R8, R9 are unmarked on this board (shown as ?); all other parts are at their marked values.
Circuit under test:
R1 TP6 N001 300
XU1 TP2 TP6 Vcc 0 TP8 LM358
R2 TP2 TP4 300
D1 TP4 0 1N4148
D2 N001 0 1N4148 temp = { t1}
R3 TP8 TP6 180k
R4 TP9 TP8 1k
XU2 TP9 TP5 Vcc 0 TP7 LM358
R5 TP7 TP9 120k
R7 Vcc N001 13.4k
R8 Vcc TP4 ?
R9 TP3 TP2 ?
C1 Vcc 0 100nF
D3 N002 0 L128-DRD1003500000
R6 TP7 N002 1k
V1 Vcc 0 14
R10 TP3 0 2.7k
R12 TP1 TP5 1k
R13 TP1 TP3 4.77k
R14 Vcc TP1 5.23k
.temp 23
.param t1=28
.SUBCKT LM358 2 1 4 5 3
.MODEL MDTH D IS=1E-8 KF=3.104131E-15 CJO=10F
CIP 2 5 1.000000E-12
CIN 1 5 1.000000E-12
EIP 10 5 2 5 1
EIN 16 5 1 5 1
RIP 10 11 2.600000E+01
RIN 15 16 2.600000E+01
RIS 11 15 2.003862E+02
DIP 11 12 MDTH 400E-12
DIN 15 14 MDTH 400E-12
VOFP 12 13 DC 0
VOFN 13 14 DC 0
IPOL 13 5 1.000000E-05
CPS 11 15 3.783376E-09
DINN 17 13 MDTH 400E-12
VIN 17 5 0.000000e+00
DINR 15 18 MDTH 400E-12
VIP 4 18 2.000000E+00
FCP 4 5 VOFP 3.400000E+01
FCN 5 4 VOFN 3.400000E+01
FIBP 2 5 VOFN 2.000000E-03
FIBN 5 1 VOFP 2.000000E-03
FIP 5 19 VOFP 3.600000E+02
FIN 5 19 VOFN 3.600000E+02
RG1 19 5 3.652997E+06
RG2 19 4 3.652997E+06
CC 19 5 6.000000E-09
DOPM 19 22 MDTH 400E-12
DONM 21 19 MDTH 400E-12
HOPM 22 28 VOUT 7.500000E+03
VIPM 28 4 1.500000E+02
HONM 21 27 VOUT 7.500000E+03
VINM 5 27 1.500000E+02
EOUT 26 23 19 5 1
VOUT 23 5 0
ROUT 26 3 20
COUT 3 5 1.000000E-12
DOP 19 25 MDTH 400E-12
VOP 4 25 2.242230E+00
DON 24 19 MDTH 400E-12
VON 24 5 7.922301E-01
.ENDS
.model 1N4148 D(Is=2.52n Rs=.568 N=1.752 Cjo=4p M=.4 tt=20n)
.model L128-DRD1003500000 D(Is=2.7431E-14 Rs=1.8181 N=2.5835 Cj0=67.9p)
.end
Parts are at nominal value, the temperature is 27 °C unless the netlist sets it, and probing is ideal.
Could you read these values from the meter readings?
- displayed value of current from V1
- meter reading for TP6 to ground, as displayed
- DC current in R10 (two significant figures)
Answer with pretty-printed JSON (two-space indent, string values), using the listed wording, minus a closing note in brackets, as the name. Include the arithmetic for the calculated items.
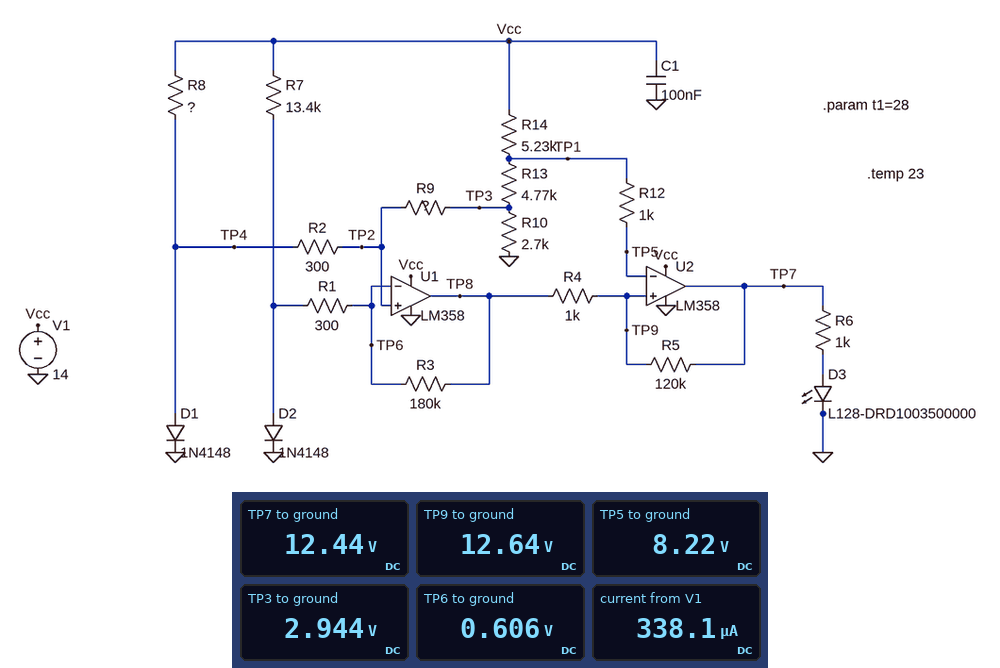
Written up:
{
  "displayed value of current from V1": "338.1 µA",
  "meter reading for TP6 to ground, as displayed": "0.606 V",
  "DC current in R10": "(2.944 V) / 2.7 kΩ = 1.1 mA"
}
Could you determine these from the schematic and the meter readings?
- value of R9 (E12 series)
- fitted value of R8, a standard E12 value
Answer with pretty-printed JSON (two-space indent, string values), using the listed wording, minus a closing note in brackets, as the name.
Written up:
{
  "value of R9": "150 kΩ",
  "fitted value of R8, a standard E12 value": "3.9 kΩ"
}
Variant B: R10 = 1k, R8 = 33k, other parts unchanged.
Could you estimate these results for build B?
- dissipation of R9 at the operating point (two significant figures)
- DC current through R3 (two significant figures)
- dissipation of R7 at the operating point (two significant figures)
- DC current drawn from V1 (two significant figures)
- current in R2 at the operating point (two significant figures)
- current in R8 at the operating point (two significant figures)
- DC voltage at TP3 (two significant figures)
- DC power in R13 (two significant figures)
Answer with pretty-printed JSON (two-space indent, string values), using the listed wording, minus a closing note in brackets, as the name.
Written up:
{
  "dissipation of R9 at the operating point": "3.4 µW",
  "DC current through R3": "3.7 µA",
  "dissipation of R7 at the operating point": "13 mW",
  "DC current drawn from V1": "3.4 mA",
  "current in R2 at the operating point": "4.8 µA",
  "current in R8 at the operating point": "410 µA",
  "DC voltage at TP3": "1.3 V",
  "DC power in R13": "7.7 mW"
}
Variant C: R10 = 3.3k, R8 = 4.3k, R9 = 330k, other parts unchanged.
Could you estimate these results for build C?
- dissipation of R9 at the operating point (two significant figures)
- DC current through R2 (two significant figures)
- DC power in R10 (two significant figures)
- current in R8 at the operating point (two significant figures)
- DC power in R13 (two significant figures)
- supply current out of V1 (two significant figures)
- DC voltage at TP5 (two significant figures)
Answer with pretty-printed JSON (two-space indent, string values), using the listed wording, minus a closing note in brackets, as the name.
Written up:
{
  "dissipation of R9 at the operating point": "24 µW",
  "DC current through R2": "8.5 µA",
  "DC power in R10": "3.6 mW",
  "current in R8 at the operating point": "3.1 mA",
  "DC power in R13": "5.3 mW",
  "supply current out of V1": "210 µA",
  "DC voltage at TP5": "8.5 V"
}
